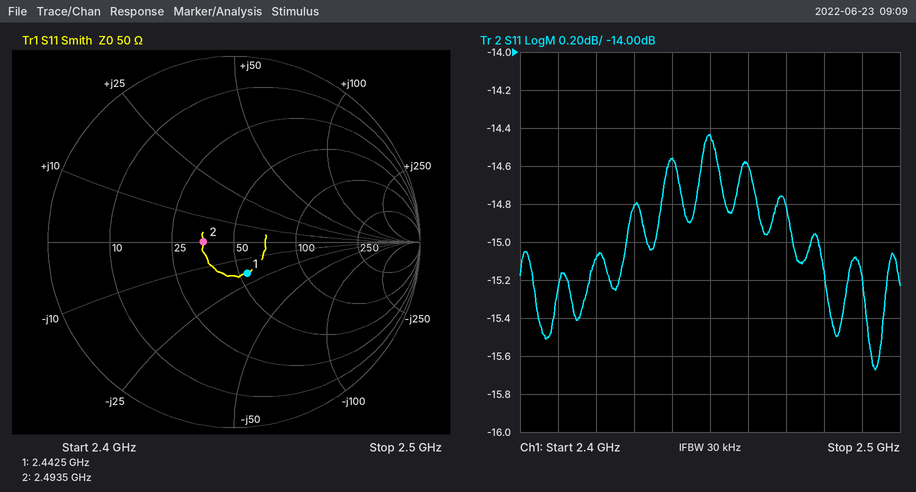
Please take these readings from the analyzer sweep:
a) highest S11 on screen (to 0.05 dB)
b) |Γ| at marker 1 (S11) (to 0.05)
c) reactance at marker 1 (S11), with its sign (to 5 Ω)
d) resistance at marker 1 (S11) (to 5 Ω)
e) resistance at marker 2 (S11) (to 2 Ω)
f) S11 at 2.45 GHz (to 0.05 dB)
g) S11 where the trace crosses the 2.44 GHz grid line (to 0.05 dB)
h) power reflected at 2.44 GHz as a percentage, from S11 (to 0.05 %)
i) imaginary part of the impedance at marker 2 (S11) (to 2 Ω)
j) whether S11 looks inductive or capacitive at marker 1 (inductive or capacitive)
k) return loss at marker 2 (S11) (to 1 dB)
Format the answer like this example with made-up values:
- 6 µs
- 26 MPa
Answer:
- -14.45 dB
- 0.20
- -20 Ω
- 55 Ω
- 36 Ω
- -14.45 dB
- -14.55 dB
- 3.50 %
- 0 Ω
- capacitive
- 16 dB
